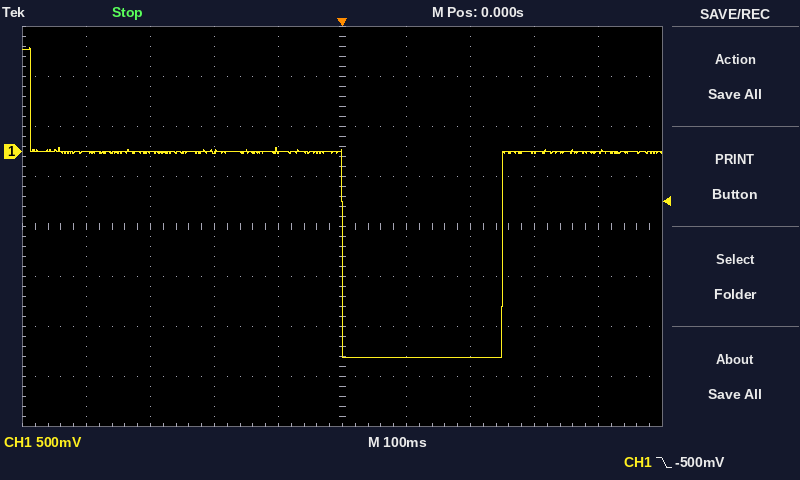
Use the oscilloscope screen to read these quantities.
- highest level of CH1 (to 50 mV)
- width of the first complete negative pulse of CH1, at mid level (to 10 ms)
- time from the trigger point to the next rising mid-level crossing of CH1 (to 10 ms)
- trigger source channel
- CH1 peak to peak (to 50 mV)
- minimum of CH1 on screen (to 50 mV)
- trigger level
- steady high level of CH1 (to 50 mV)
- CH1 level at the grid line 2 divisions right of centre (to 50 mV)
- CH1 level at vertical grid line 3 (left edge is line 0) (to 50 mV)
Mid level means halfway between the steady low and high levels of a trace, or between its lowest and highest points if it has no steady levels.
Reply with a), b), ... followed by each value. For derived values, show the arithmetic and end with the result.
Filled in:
a) 1.05 V
b) 250 ms
c) 250 ms
d) CH1
e) 1.05 V − (-2.05 V) = 3.10 V
f) -2.05 V
g) -500 mV
h) 0 mV
i) -2.05 V
j) 0 mV
